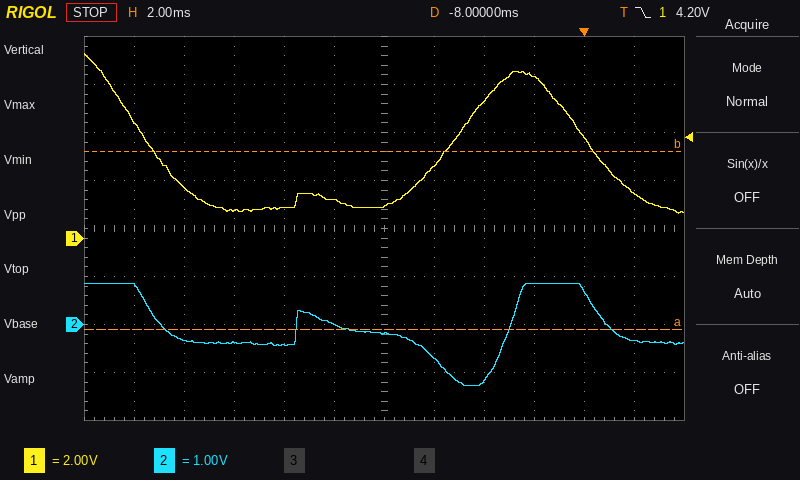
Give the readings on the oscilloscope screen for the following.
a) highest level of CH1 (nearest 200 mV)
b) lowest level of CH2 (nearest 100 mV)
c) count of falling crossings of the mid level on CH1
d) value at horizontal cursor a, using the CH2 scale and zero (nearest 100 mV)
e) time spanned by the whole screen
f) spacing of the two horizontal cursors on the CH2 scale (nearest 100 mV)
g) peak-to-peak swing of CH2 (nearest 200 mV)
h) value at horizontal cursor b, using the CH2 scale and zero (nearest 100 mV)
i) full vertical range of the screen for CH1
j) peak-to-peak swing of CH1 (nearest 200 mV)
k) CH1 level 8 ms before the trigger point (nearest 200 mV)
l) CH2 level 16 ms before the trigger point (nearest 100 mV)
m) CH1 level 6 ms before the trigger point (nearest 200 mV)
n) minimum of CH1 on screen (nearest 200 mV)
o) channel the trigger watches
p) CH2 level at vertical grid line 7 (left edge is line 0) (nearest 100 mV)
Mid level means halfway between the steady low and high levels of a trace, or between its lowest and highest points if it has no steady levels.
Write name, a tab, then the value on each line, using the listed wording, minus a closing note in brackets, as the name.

highest level of CH1	7.6 V
lowest level of CH2	-1.3 V
count of falling crossings of the mid level on CH1	2
value at horizontal cursor a, using the CH2 scale and zero	-100 mV
time spanned by the whole screen	24 ms
spacing of the two horizontal cursors on the CH2 scale	3.7 V
peak-to-peak swing of CH2	2.2 V
value at horizontal cursor b, using the CH2 scale and zero	3.6 V
full vertical range of the screen for CH1	16 V
peak-to-peak swing of CH1	6.6 V
CH1 level 8 ms before the trigger point	1.4 V
CH2 level 16 ms before the trigger point	-300 mV
CH1 level 6 ms before the trigger point	3.0 V
minimum of CH1 on screen	1.0 V
channel the trigger watches	CH1
CH2 level at vertical grid line 7 (left edge is line 0)	-700 mV
